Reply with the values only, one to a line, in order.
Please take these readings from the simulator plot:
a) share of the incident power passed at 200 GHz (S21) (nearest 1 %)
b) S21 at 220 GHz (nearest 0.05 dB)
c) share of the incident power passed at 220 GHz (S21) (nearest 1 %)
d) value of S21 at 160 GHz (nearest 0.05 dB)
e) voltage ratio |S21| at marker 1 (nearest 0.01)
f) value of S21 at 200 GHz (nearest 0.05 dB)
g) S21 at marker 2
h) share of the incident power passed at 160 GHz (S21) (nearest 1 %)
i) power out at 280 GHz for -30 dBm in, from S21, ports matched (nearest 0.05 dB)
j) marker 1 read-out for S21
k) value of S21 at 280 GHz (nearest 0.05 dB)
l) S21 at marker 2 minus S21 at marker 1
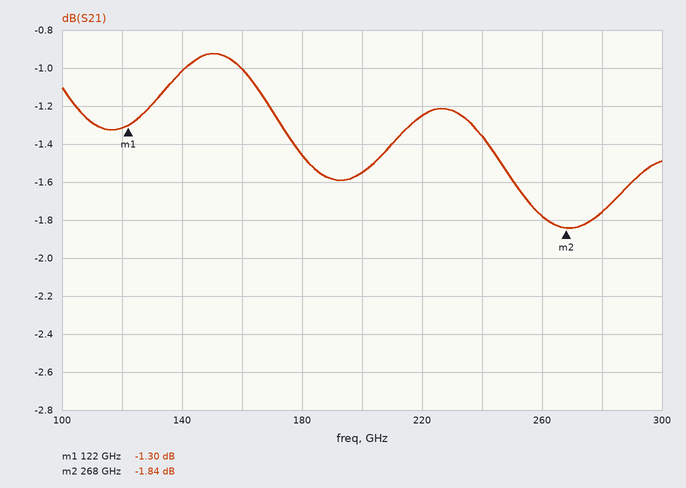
70 %
-1.25 dB
75 %
-1.00 dB
0.86
-1.55 dB
-1.84 dB
79 %
-31.75 dBm
-1.30 dB
-1.75 dB
-0.54 dB
